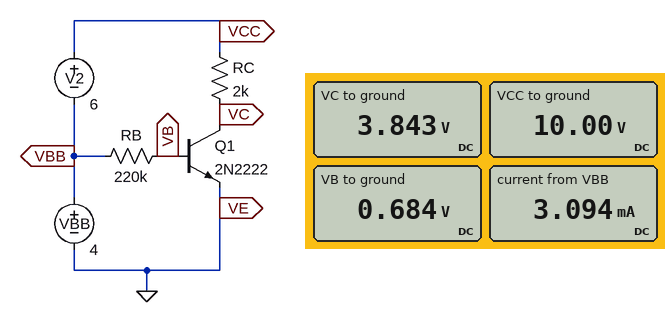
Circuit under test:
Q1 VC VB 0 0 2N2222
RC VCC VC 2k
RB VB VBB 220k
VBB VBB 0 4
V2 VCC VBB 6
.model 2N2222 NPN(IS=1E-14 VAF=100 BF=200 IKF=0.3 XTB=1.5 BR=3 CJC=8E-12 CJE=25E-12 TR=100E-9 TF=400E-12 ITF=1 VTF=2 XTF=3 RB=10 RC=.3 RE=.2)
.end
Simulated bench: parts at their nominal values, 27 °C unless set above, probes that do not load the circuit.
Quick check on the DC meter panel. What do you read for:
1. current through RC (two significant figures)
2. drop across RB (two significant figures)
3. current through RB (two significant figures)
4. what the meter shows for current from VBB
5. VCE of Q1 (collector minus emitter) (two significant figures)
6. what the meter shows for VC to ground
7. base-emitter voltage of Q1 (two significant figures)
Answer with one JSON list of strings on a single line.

["3.1 mA", "3.3 V", "15 µA", "3.094 mA", "3.8 V", "3.843 V", "680 mV"]
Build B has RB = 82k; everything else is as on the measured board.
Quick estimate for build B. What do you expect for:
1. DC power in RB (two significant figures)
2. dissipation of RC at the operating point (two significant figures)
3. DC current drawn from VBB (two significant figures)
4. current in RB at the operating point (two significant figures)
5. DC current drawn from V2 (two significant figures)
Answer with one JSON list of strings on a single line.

["130 µW", "49 mW", "5.0 mA", "40 µA", "4.9 mA"]
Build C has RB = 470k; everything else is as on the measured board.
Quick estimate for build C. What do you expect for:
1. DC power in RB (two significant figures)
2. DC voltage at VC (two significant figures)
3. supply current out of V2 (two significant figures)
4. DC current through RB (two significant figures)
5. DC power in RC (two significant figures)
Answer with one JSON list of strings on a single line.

["24 µW", "7.0 V", "1.5 mA", "7.1 µA", "4.5 mW"]
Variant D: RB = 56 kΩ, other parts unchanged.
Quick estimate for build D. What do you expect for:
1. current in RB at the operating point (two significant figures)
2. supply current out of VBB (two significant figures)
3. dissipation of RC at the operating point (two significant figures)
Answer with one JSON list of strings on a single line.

["59 µA", "5.0 mA", "49 mW"]
